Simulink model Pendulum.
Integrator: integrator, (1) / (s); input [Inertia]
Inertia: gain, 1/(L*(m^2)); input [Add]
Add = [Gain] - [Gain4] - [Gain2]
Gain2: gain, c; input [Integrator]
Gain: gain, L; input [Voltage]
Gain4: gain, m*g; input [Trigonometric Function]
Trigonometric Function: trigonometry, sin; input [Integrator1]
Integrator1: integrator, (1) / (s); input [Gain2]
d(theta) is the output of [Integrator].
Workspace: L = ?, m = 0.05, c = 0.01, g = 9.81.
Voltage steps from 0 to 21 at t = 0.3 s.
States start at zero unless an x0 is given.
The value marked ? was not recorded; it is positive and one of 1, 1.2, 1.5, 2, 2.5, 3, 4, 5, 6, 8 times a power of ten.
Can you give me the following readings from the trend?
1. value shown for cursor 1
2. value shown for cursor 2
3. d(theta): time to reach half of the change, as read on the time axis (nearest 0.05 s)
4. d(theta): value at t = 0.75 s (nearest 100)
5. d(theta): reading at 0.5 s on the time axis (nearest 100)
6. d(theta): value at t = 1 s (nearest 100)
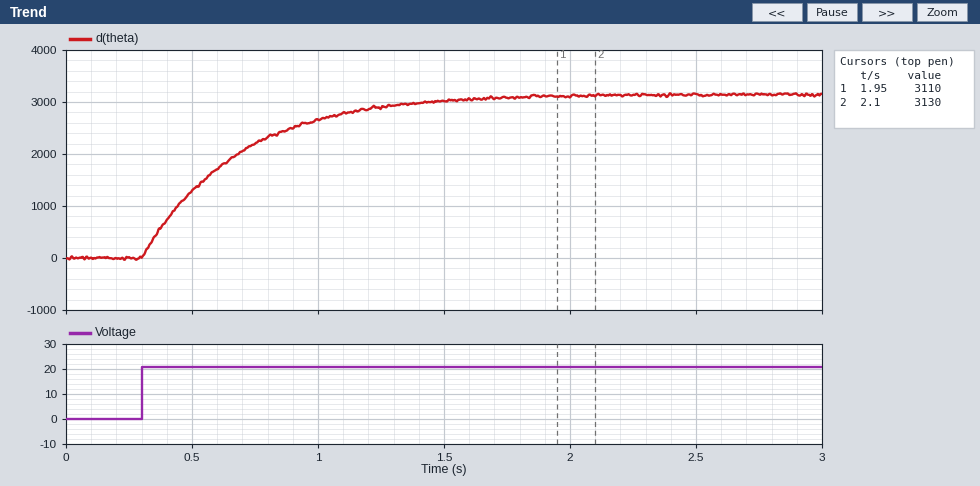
3110
3130
0.55 s
2200
1300
2700
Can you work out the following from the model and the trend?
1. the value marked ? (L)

1.5
